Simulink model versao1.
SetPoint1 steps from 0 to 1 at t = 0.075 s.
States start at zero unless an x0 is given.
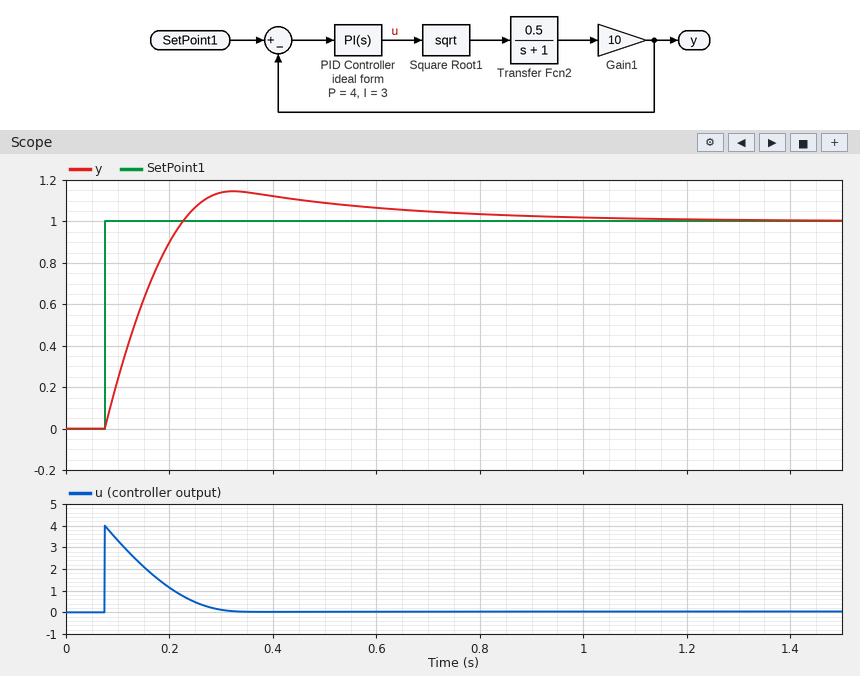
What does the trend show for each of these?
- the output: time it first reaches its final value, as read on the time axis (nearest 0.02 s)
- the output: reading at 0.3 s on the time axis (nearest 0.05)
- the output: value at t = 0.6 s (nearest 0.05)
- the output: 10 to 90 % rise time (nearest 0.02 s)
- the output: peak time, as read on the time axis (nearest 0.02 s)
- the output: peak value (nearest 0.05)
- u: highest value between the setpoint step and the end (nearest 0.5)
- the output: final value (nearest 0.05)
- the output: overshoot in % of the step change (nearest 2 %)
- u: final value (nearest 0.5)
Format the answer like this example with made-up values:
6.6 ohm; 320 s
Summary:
0.22 s; 1.15; 1.05; 0.12 s; 0.32 s; 1.15; 4.0; 1.00; 14 %; 0.0
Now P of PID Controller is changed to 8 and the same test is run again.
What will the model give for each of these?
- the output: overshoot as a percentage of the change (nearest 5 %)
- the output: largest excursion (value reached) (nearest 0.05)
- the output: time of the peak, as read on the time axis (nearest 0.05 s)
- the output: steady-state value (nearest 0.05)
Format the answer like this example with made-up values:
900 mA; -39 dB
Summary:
10 %; 1.10; 0.25 s; 1.00
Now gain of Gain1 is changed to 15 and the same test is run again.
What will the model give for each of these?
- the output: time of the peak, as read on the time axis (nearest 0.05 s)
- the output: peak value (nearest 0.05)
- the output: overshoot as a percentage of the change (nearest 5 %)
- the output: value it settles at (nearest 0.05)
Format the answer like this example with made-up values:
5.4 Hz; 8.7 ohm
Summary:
0.25 s; 1.10; 10 %; 1.00
